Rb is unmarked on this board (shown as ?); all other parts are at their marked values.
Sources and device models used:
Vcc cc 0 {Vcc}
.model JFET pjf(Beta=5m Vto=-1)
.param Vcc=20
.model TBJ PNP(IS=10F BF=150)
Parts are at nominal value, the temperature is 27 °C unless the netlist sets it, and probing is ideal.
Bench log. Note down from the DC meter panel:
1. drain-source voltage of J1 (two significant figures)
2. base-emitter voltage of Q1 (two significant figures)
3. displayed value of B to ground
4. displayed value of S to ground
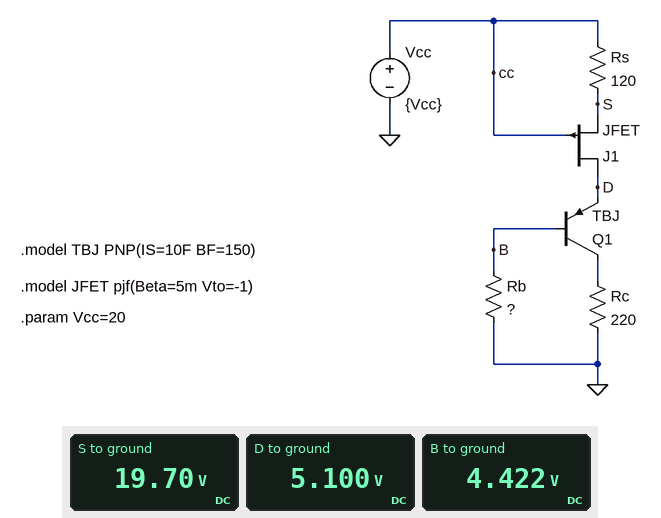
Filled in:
-15 V
-680 mV
4.422 V
19.70 V
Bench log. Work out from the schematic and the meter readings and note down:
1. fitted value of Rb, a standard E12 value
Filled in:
270 kΩ
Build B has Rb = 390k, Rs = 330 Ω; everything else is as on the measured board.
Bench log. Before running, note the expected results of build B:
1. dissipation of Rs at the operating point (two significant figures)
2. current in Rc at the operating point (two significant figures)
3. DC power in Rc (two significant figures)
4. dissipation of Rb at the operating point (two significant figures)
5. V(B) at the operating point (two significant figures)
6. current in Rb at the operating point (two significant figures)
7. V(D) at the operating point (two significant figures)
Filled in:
660 µW
1.4 mA
440 µW
34 µW
3.7 V
9.4 µA
4.3 V
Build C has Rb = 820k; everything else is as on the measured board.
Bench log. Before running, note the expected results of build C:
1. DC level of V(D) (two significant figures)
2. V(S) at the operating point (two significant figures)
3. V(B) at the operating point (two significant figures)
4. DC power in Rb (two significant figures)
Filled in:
14 V
20 V
13 V
220 µW
